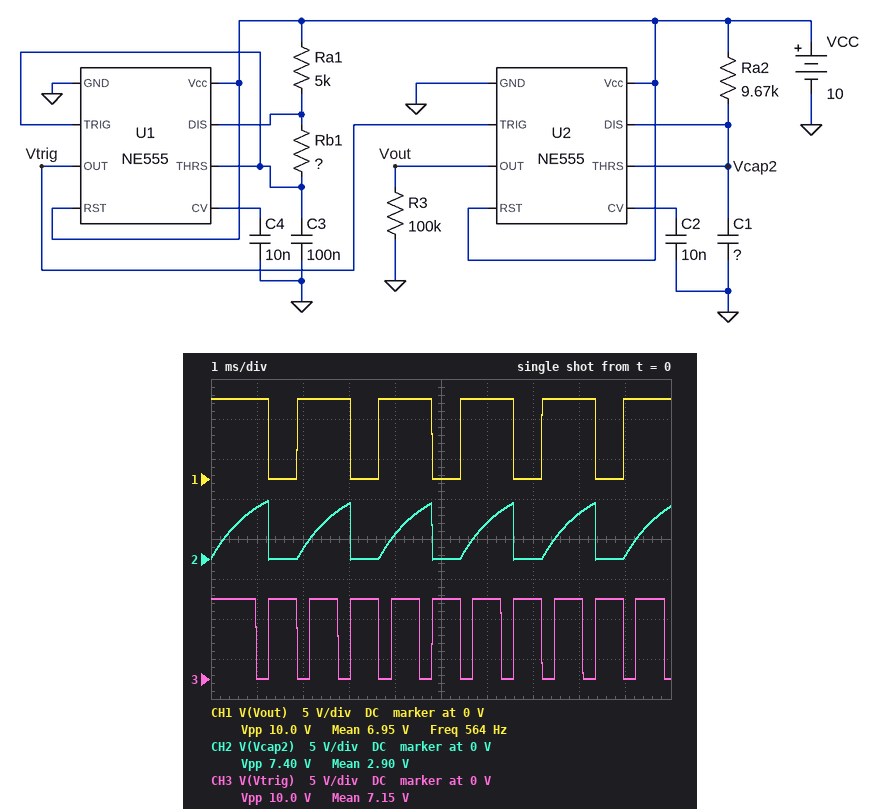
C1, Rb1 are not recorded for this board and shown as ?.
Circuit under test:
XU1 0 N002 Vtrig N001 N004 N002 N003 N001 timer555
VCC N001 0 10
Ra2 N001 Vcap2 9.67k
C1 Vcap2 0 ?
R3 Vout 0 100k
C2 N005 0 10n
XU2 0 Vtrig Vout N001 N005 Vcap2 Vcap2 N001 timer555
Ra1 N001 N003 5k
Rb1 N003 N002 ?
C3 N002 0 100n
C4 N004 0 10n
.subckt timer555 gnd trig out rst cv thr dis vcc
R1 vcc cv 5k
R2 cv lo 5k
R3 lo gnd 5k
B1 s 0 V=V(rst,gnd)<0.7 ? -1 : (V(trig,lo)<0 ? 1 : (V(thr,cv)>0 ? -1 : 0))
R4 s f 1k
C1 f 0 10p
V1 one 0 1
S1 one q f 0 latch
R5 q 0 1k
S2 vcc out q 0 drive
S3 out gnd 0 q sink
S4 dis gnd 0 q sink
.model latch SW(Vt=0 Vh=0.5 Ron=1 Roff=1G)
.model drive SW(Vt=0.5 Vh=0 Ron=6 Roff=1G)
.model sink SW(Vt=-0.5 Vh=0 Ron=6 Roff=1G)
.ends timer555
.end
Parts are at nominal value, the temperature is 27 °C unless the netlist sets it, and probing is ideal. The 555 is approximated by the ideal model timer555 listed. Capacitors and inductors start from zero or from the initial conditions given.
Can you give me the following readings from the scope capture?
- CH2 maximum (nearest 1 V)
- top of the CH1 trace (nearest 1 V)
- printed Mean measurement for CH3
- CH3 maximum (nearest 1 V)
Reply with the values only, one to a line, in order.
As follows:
7 V
10 V
7.15 V
10 V
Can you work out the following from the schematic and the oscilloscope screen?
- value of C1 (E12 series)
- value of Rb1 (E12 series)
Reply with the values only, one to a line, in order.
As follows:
100 nF
3.9 kΩ
